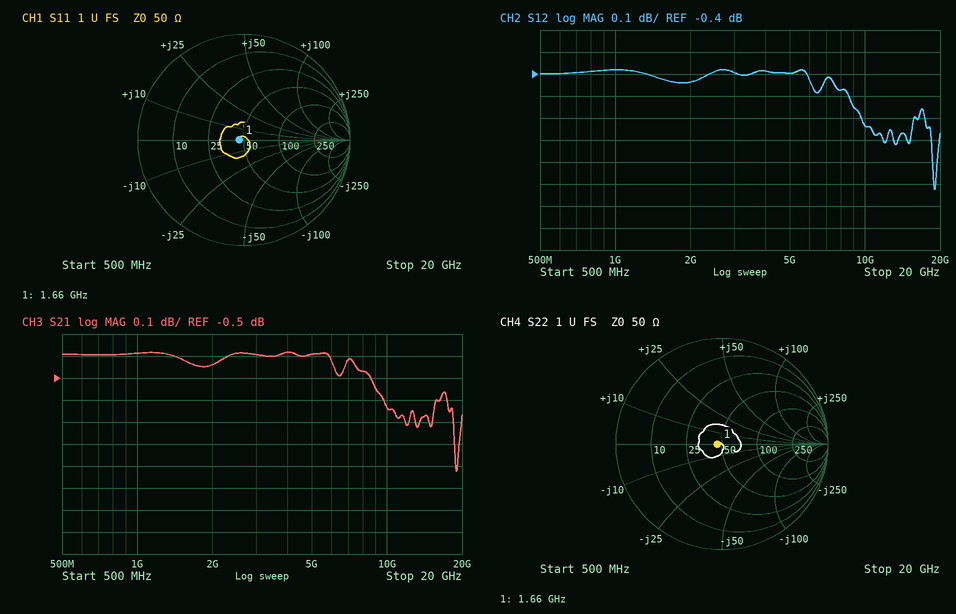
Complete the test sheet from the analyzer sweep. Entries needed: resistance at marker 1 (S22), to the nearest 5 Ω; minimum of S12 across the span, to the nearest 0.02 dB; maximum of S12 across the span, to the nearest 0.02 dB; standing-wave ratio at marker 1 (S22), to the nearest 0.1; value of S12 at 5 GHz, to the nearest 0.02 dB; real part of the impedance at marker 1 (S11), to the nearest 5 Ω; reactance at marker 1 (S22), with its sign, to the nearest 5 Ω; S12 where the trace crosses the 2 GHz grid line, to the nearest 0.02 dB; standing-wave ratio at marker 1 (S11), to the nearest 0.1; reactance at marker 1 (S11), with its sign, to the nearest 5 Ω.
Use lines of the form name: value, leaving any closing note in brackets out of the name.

resistance at marker 1 (S22), to the nearest 5 Ω: 45 Ω
minimum of S12 across the span, to the nearest 0.02 dB: -0.92 dB
maximum of S12 across the span, to the nearest 0.02 dB: -0.38 dB
standing-wave ratio at marker 1 (S22), to the nearest 0.1: 1.1
value of S12 at 5 GHz, to the nearest 0.02 dB: -0.40 dB
real part of the impedance at marker 1 (S11), to the nearest 5 Ω: 45 Ω
reactance at marker 1 (S22), with its sign, to the nearest 5 Ω: 0 Ω
S12 where the trace crosses the 2 GHz grid line, to the nearest 0.02 dB: -0.44 dB
standing-wave ratio at marker 1 (S11), to the nearest 0.1: 1.1
reactance at marker 1 (S11), with its sign, to the nearest 5 Ω: 0 Ω
